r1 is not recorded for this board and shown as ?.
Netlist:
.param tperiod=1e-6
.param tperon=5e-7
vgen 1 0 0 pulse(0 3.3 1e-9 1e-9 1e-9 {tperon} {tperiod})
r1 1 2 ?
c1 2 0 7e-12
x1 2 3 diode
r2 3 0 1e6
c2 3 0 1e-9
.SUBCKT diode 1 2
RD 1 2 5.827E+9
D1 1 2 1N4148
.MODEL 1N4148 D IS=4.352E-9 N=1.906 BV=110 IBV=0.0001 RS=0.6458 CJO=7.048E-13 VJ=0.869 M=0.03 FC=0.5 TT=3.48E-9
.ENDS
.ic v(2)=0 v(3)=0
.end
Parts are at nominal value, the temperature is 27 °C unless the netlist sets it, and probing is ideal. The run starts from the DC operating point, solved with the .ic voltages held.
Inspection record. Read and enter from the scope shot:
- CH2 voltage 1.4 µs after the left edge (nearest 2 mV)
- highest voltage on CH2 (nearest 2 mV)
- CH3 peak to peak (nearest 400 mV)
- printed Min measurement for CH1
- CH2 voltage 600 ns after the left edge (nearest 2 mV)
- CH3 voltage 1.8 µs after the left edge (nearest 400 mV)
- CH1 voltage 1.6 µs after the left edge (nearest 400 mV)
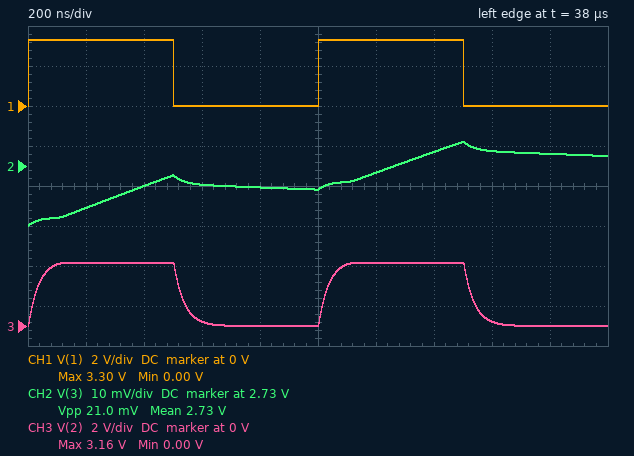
2.734 V
2.736 V
3.2 V
0.00 V
2.726 V
0 V
0 V
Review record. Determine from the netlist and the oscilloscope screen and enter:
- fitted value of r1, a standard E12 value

4.7 kΩ
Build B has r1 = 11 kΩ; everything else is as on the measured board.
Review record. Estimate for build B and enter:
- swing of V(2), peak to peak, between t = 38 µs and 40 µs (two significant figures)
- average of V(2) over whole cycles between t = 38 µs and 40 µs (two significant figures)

2.6 V
1.4 V
